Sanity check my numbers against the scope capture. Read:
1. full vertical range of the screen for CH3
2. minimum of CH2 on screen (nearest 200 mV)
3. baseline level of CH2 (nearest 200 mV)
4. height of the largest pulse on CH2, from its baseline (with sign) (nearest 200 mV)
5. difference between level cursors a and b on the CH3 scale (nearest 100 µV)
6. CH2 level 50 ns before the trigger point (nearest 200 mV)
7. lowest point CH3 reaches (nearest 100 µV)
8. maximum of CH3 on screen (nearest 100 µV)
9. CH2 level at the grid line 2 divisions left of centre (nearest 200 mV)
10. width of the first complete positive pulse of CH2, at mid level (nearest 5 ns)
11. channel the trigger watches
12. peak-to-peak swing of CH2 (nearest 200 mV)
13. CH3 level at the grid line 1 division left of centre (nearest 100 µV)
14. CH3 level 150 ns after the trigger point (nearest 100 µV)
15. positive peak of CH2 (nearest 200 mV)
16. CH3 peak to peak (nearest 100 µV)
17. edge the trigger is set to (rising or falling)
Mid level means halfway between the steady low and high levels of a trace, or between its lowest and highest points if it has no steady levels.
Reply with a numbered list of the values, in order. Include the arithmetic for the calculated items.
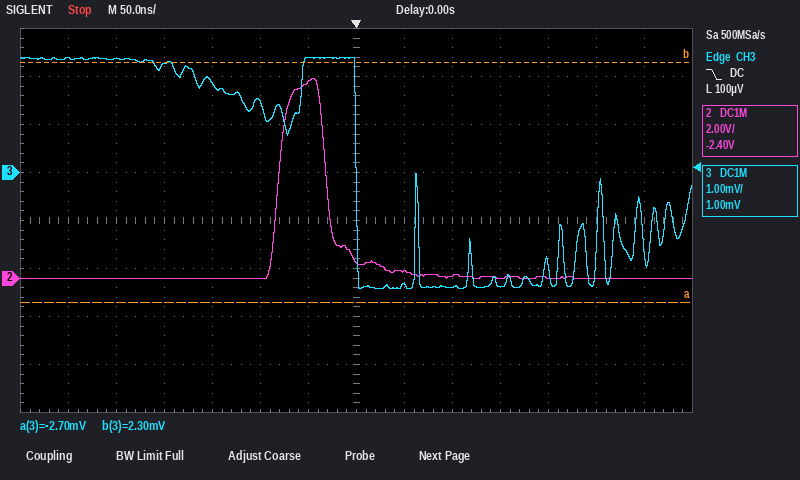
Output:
1. 8 mV
2. 0.0 V
3. 0.0 V
4. 8.4 V − (0.0 V) = +8.4 V
5. 5.0 mV
6. 8.2 V
7. -2.4 mV
8. 2.4 mV
9. 0.0 V
10. 50 ns
11. CH3
12. 8.4 V − (0.0 V) = 8.4 V
13. 2.4 mV
14. -2.4 mV
15. 8.4 V
16. 2.4 mV − (-2.4 mV) = 4.8 mV
17. falling
